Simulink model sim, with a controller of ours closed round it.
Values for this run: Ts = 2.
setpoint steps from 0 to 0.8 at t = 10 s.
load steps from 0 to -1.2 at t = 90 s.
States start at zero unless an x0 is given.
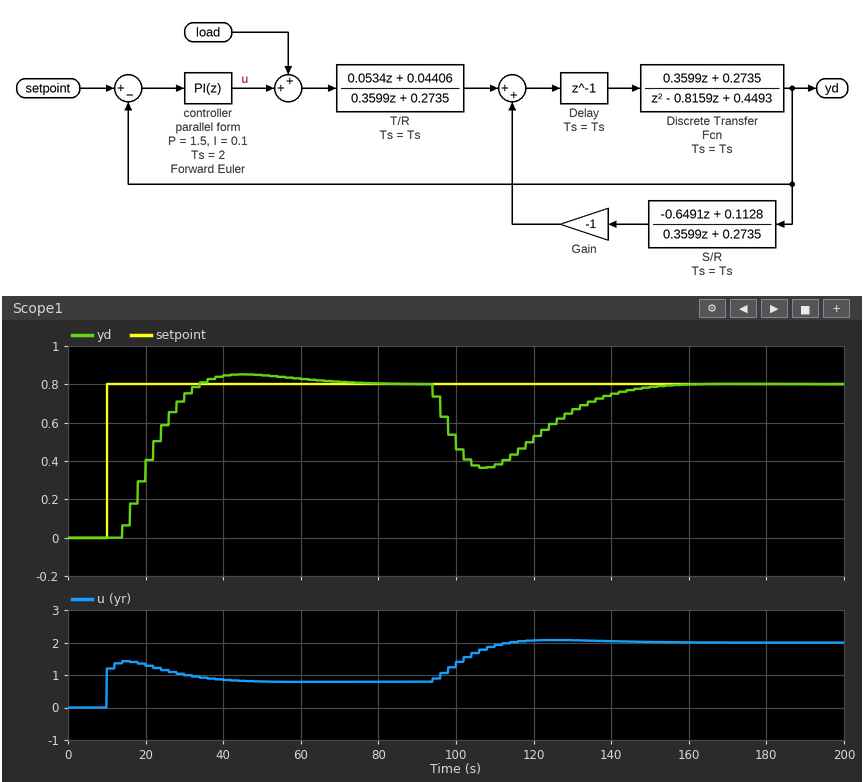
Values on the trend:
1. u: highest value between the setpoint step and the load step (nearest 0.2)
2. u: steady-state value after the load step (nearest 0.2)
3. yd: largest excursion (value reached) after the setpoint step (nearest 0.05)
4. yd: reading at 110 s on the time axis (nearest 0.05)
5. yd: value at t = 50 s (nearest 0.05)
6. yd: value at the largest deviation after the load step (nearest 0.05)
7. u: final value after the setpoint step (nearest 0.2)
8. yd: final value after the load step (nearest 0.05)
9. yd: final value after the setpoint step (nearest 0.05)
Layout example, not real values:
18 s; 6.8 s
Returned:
1.4; 2.0; 0.85; 0.40; 0.85; 0.35; 0.8; 0.80; 0.80
